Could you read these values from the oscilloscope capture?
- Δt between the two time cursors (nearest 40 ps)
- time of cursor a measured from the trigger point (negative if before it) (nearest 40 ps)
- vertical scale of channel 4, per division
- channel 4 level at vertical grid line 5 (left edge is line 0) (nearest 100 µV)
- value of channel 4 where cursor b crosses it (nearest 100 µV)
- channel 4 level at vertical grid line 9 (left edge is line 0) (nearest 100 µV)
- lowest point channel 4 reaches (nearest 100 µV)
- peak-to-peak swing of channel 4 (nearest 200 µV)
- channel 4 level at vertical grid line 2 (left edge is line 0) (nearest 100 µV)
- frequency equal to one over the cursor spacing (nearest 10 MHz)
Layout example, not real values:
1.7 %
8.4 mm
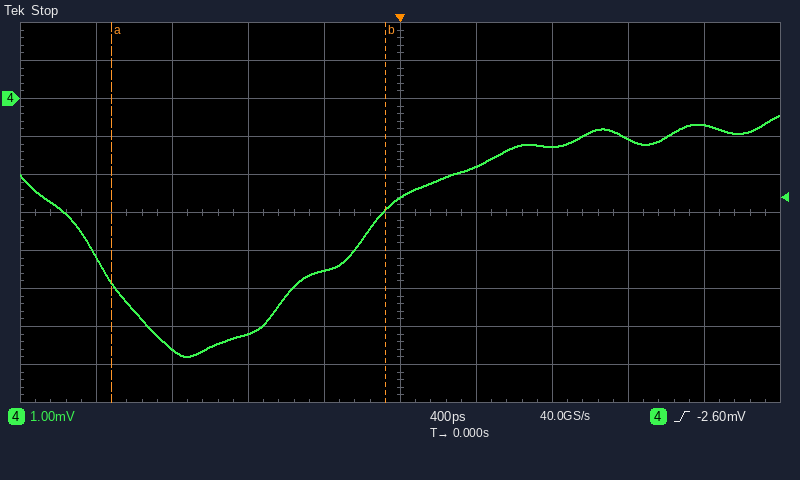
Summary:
1.44 ns
-1.52 ns
1 mV
-2.6 mV
-2.9 mV
-700 µV
-6.8 mV
6.4 mV
-6.6 mV
690 MHz
